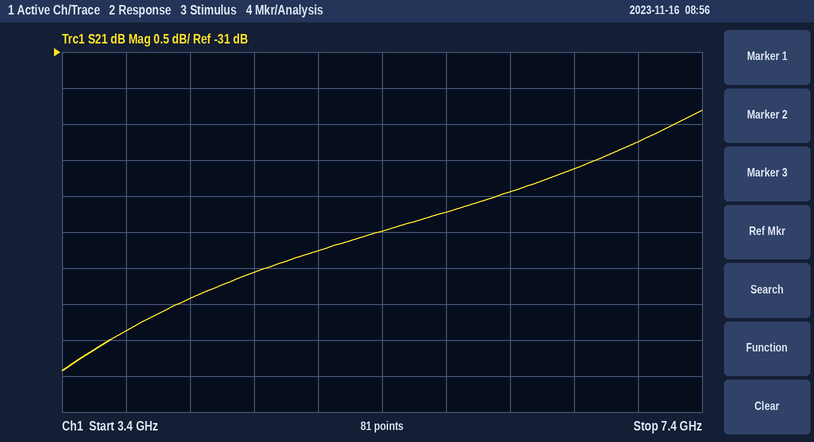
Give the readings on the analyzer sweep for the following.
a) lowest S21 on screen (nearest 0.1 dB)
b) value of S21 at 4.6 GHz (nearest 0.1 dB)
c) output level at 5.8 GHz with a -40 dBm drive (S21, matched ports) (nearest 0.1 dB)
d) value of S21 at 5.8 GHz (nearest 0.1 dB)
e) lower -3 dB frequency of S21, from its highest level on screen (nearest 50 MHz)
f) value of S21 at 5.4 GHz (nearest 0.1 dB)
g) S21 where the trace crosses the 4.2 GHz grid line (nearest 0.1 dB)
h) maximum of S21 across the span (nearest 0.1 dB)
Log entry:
-35.4 dB
-34.1 dB
-73.2 dBm
-33.2 dB
3.85 GHz
-33.5 dB
-34.4 dB
-31.8 dB
